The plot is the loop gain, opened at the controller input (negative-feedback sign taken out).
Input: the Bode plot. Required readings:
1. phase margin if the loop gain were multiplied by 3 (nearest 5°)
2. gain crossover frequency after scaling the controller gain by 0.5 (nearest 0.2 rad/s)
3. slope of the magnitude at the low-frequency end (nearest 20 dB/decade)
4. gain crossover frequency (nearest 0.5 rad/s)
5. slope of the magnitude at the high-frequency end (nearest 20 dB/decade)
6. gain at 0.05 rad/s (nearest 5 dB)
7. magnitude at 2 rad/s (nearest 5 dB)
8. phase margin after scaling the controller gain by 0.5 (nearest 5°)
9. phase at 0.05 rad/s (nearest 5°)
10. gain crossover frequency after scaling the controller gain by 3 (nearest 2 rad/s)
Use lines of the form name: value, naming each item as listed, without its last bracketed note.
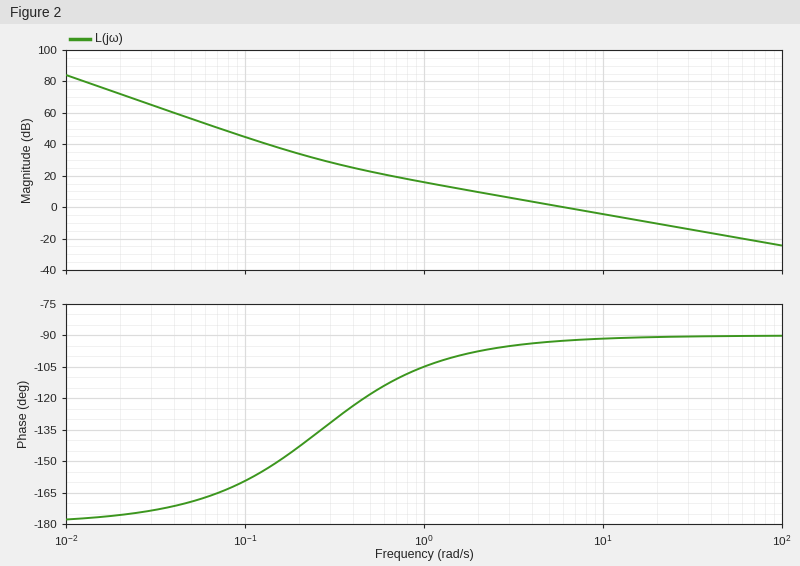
phase margin if the loop gain were multiplied by 3: 90°
gain crossover frequency after scaling the controller gain by 0.5: 3.0 rad/s
slope of the magnitude at the low-frequency end: -40 dB/decade
gain crossover frequency: 6.0 rad/s
slope of the magnitude at the high-frequency end: -20 dB/decade
gain at 0.05 rad/s: 55 dB
magnitude at 2 rad/s: 10 dB
phase margin after scaling the controller gain by 0.5: 85°
phase at 0.05 rad/s: -170°
gain crossover frequency after scaling the controller gain by 3: 18 rad/s
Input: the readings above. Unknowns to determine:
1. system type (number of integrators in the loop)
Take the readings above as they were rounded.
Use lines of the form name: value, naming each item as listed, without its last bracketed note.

system type: 2
